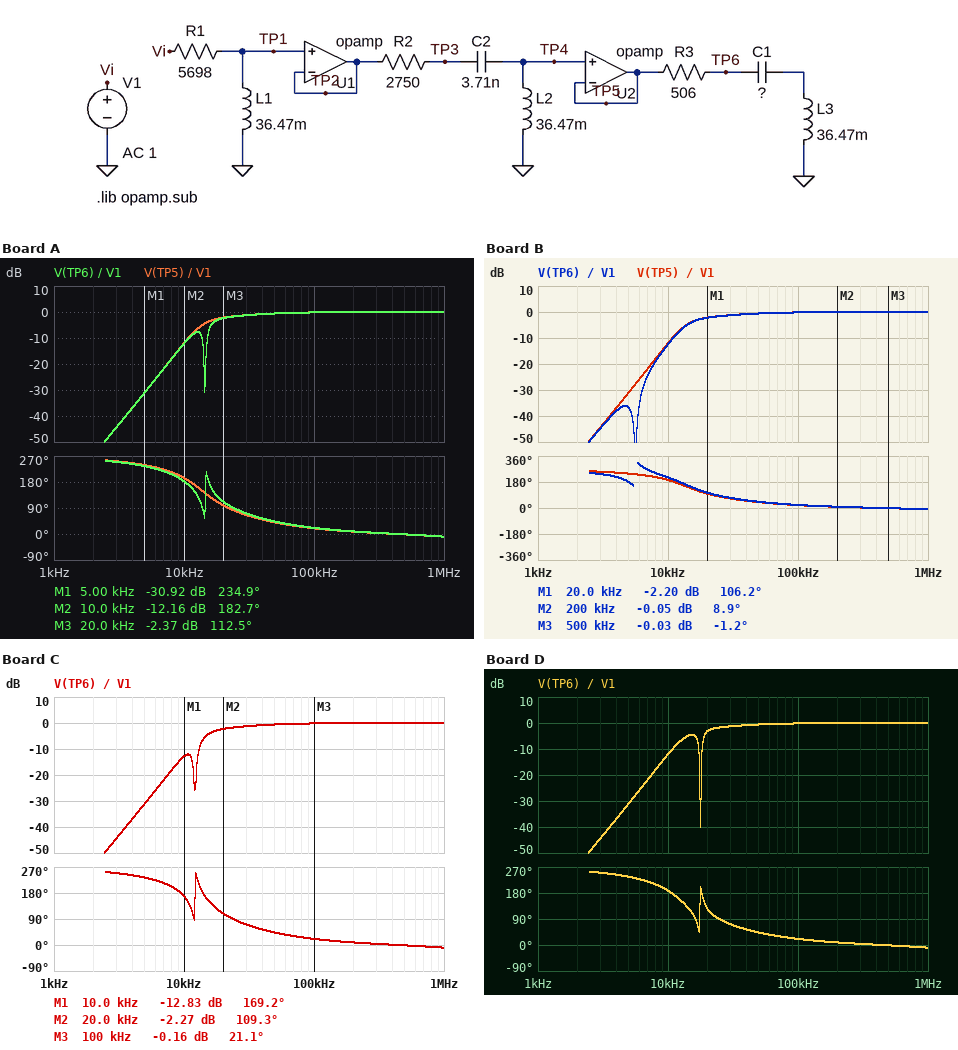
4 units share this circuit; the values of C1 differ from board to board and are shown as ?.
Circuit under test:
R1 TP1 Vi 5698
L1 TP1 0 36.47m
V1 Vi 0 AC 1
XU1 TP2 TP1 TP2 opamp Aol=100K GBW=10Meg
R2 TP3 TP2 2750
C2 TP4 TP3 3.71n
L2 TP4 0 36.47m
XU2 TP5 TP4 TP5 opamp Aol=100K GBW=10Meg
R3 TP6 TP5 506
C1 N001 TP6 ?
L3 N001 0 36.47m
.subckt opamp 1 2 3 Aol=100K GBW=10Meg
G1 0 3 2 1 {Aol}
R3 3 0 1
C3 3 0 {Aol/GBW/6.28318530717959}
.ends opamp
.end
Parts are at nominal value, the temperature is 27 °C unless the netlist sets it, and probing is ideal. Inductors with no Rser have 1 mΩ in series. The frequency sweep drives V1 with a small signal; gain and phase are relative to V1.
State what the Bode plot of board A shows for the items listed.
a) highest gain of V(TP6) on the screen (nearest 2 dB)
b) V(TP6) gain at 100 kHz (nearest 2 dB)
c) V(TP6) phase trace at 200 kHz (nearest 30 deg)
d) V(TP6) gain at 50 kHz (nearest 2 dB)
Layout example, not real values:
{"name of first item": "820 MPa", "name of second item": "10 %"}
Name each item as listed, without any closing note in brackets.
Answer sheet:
{"highest gain of V(TP6) on the screen": "0 dB", "V(TP6) gain at 100 kHz": "0 dB", "V(TP6) phase trace at 200 kHz": "0 deg", "V(TP6) gain at 50 kHz": "0 dB"}
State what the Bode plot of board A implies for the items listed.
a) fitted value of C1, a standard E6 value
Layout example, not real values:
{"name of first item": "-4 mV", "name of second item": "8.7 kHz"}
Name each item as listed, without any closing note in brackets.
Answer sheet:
{"fitted value of C1, a standard E6 value": "3.3 nF"}
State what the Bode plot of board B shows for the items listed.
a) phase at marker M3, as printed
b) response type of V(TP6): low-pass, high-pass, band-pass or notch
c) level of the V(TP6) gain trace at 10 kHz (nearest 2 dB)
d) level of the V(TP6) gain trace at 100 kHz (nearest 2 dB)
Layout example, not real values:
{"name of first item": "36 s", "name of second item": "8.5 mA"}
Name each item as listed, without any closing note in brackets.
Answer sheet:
{"phase at marker M3, as printed": "-1.2 deg", "response type of V(TP6): low-pass, high-pass, band-pass or notch": "high-pass", "level of the V(TP6) gain trace at 10 kHz": "-12 dB", "level of the V(TP6) gain trace at 100 kHz": "0 dB"}
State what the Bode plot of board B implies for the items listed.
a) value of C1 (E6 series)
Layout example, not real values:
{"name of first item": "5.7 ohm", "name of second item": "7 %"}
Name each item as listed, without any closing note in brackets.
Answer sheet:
{"value of C1": "22 nF"}
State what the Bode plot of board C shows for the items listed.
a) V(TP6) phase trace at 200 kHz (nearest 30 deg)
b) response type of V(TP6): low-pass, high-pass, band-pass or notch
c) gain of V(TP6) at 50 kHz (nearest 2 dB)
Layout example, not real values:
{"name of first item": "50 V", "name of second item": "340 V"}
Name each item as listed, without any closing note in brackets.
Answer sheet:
{"V(TP6) phase trace at 200 kHz": "0 deg", "response type of V(TP6): low-pass, high-pass, band-pass or notch": "high-pass", "gain of V(TP6) at 50 kHz": "0 dB"}
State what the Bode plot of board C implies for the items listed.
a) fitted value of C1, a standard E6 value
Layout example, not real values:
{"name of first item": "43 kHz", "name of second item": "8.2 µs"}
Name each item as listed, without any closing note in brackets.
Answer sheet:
{"fitted value of C1, a standard E6 value": "4.7 nF"}
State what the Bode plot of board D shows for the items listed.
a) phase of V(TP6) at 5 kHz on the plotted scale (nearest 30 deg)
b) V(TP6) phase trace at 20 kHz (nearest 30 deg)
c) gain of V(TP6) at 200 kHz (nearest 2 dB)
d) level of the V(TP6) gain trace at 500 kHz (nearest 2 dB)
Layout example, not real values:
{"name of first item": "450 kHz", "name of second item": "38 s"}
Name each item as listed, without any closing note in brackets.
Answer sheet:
{"phase of V(TP6) at 5 kHz on the plotted scale": "240 deg", "V(TP6) phase trace at 20 kHz": "120 deg", "gain of V(TP6) at 200 kHz": "0 dB", "level of the V(TP6) gain trace at 500 kHz": "0 dB"}
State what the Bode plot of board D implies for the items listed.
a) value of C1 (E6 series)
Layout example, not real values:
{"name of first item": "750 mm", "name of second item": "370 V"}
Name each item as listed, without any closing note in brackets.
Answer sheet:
{"value of C1": "2.2 nF"}
